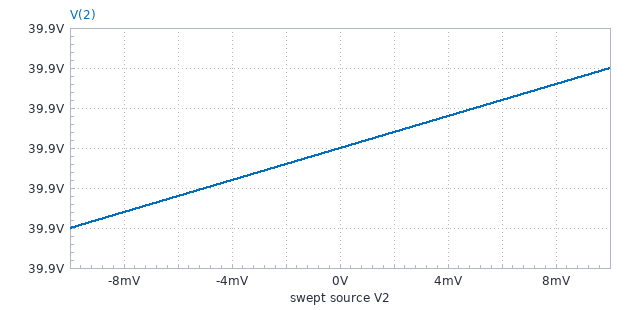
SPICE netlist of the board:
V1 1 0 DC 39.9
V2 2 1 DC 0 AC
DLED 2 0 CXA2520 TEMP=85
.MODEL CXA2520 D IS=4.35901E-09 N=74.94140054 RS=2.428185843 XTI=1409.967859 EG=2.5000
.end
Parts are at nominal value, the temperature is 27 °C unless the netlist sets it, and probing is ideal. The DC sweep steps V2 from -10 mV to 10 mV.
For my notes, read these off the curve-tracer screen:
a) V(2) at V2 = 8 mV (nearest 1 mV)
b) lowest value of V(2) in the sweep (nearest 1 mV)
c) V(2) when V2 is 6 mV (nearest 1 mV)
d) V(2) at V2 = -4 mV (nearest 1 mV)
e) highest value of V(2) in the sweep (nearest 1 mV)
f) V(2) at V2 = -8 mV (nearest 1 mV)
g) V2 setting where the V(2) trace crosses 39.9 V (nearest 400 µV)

39.908 V
39.890 V
39.906 V
39.896 V
39.910 V
39.892 V
0 V
